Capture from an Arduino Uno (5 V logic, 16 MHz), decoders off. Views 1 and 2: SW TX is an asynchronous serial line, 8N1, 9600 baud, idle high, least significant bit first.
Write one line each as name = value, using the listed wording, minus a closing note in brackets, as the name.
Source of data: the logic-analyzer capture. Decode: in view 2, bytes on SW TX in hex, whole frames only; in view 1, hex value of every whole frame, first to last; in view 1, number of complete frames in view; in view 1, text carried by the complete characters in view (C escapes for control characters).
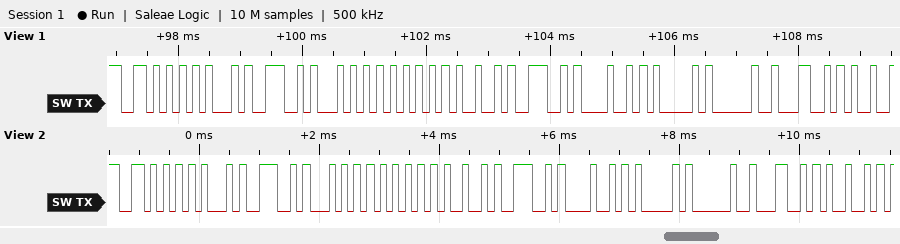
in view 2, bytes on SW TX in hex, whole frames only = 56 45 4E 54 55 49 4E 48 41 20 4C 49
in view 1, hex value of every whole frame, first to last = 56 45 4E 54 55 49 4E 48 41 20 4C
in view 1, number of complete frames in view = 11
in view 1, text carried by the complete characters in view = "VENTUINHA L"
